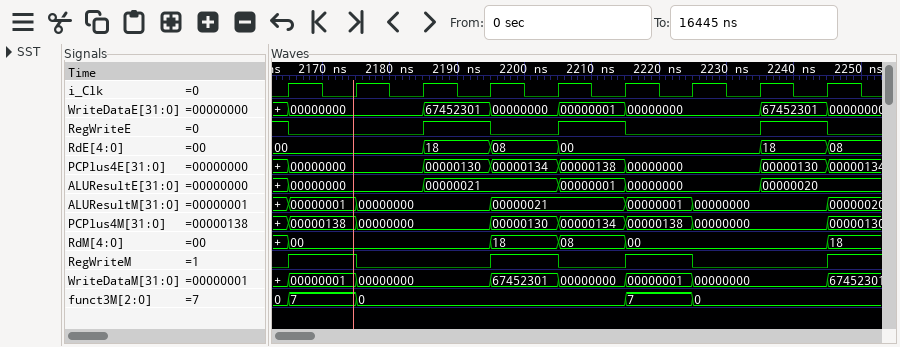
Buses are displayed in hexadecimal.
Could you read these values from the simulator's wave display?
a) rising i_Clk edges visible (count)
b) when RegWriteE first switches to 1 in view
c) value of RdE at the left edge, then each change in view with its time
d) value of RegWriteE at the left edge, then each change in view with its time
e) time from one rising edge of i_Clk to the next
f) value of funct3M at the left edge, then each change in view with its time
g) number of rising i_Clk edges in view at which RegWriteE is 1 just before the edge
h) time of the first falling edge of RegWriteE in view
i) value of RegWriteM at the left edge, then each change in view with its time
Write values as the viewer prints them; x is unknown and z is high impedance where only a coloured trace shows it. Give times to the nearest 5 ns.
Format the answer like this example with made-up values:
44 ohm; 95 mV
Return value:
9; 2185 ns; 00, 18 at 2185 ns, 08 at 2195 ns, 00 at 2205 ns, 18 at 2235 ns, 08 at 2245 ns; 1, 0 at 2165 ns, 1 at 2185 ns, 0 at 2195 ns, 1 at 2205 ns, 0 at 2215 ns, 1 at 2235 ns, 0 at 2245 ns; 10 ns; 0, 7 at 2165 ns, 0 at 2175 ns, 7 at 2215 ns, 0 at 2225 ns; 4; 2165 ns; 0, 1 at 2165 ns, 0 at 2175 ns, 1 at 2195 ns, 0 at 2205 ns, 1 at 2215 ns, 0 at 2225 ns, 1 at 2245 ns
